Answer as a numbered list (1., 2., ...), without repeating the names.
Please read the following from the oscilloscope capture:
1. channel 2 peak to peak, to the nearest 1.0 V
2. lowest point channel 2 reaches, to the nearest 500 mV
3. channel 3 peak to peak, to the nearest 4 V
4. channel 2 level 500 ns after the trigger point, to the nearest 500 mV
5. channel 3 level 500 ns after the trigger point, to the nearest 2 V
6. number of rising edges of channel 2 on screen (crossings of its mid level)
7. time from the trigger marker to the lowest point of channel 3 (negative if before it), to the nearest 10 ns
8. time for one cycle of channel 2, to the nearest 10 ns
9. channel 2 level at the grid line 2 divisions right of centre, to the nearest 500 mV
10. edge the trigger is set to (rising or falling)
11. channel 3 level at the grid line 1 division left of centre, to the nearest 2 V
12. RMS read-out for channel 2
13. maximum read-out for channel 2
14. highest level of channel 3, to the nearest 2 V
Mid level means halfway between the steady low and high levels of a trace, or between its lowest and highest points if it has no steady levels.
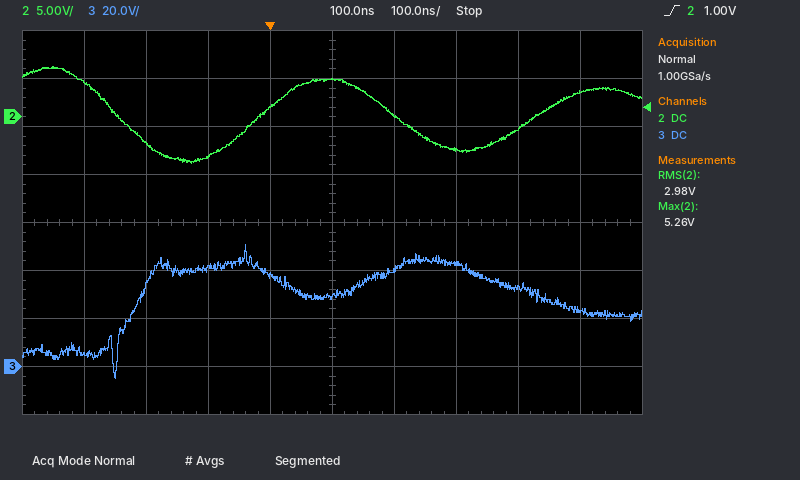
1. 10.0 V
2. -5.0 V
3. 56 V
4. 2.5 V
5. 24 V
6. 2
7. -250 ns
8. 450 ns
9. -3.5 V
10. rising
11. 38 V
12. 2.98 V
13. 5.26 V
14. 50 V
